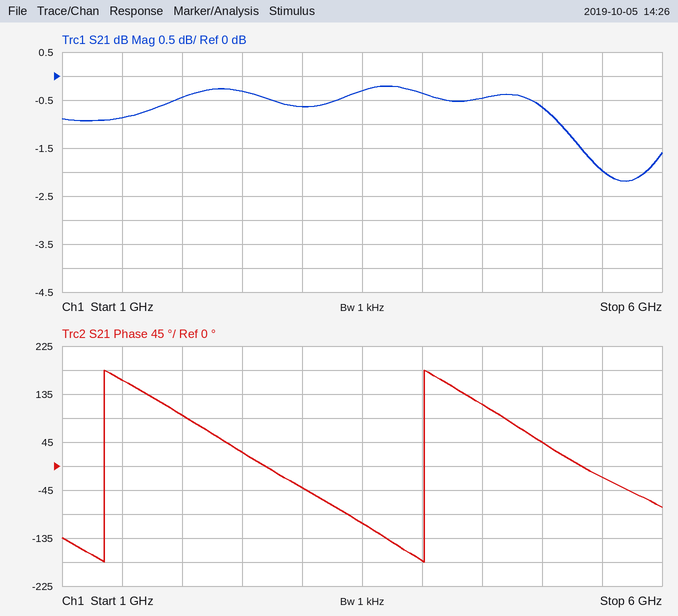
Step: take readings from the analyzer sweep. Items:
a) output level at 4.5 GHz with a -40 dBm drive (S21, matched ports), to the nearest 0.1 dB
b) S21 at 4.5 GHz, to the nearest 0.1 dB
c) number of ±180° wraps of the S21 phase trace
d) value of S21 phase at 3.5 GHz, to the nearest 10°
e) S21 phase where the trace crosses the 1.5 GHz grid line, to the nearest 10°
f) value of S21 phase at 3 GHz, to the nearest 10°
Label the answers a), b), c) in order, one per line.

a) -40.5 dBm
b) -0.5 dB
c) 2
d) -110°
e) 160°
f) -40°
